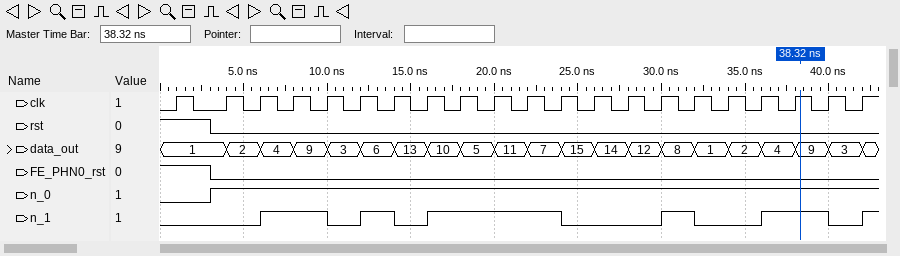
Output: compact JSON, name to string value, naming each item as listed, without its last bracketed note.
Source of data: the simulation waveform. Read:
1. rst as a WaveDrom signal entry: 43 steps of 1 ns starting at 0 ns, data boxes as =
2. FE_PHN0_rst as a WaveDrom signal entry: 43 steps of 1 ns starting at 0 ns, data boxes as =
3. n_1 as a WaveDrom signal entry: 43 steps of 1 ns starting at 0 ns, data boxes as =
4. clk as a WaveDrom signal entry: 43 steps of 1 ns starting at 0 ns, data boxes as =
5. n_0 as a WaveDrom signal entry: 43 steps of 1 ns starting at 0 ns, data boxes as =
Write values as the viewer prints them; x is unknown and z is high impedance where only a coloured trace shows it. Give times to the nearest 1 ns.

{"rst as a WaveDrom signal entry: 43 steps of 1 ns starting at 0 ns, data boxes as =": "{name: 'rst', wave: '1..0.......................................'}", "FE_PHN0_rst as a WaveDrom signal entry: 43 steps of 1 ns starting at 0 ns, data boxes as =": "{name: 'FE_PHN0_rst', wave: '1..0.......................................'}", "n_1 as a WaveDrom signal entry: 43 steps of 1 ns starting at 0 ns, data boxes as =": "{name: 'n_1', wave: '0.....1...0.1.0.1.......0.....1.0...1...0.1'}", "clk as a WaveDrom signal entry: 43 steps of 1 ns starting at 0 ns, data boxes as =": "{name: 'clk', wave: '010.101010101010101010101010101010101010101'}", "n_0 as a WaveDrom signal entry: 43 steps of 1 ns starting at 0 ns, data boxes as =": "{name: 'n_0', wave: '0..1.......................................'}"}
